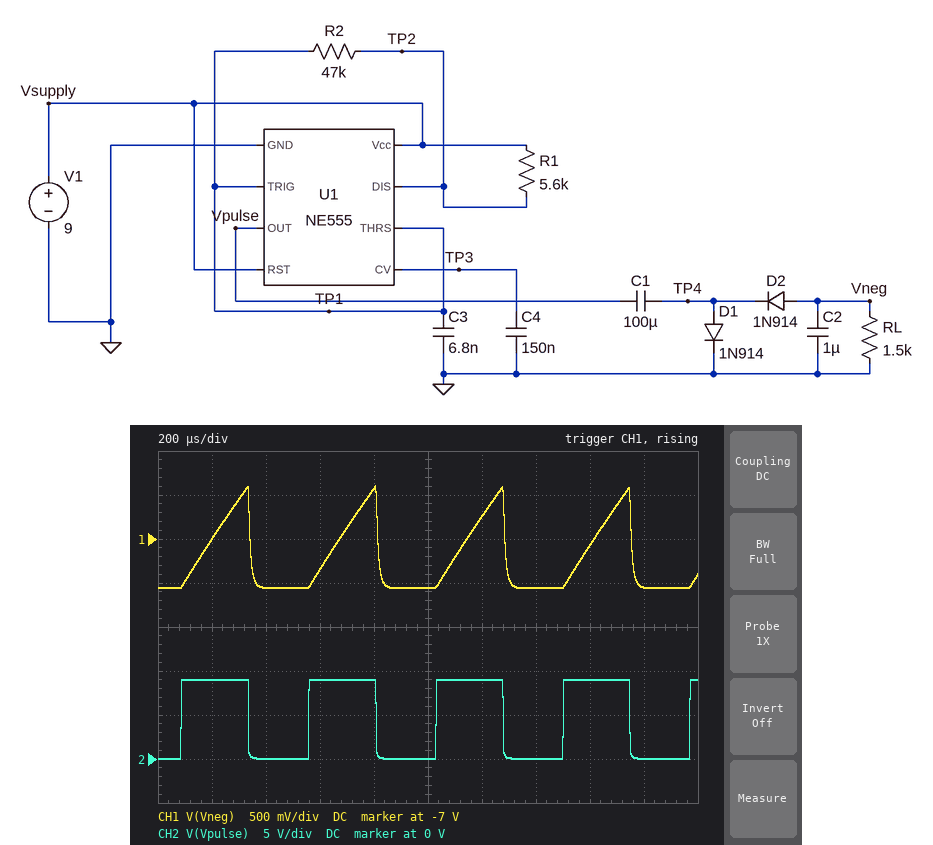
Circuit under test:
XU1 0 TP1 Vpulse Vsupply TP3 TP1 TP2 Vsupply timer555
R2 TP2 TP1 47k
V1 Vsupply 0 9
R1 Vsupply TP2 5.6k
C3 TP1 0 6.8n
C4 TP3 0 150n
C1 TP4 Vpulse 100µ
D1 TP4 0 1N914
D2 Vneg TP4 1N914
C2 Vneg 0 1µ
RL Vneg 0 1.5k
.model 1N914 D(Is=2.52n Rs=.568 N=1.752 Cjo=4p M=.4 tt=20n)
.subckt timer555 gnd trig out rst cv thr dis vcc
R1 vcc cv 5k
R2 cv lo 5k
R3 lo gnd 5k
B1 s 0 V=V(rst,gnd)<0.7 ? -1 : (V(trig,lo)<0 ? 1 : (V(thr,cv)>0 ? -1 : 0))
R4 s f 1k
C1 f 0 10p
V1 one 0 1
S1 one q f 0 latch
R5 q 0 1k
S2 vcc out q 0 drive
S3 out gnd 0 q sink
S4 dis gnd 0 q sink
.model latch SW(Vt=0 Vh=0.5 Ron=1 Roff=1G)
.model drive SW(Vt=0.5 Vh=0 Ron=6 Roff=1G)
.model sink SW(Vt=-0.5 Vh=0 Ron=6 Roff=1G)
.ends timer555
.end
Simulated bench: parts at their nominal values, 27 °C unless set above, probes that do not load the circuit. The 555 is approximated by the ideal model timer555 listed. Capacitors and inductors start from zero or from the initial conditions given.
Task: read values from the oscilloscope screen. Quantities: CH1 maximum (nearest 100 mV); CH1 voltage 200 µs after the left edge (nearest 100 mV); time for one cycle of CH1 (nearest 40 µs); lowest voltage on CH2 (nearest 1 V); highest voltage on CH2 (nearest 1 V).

-6.4 V
-7.0 V
480 µs
0 V
9 V
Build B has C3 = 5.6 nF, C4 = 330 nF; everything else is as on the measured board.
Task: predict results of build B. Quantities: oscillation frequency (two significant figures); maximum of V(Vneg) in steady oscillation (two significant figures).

2.6 kHz
-6.6 V
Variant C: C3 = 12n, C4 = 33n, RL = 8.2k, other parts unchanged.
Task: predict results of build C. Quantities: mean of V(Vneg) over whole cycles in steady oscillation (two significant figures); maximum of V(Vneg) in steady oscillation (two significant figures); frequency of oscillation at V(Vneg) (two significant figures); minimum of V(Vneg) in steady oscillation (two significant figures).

-7.7 V
-7.4 V
1.2 kHz
-7.8 V
